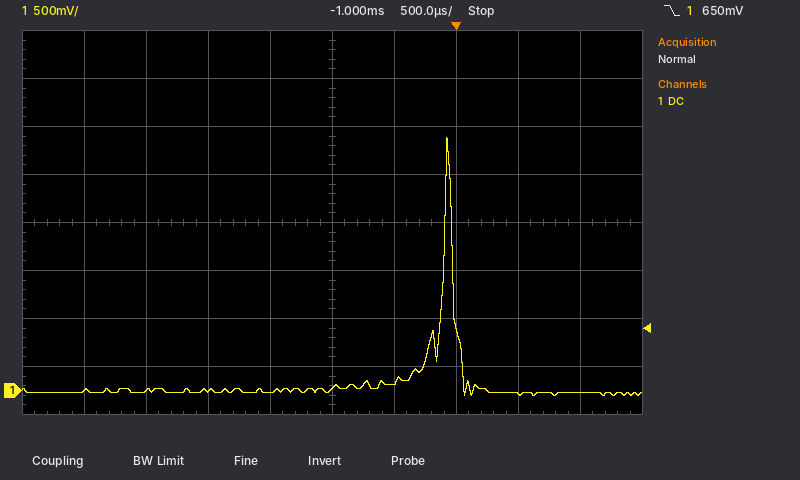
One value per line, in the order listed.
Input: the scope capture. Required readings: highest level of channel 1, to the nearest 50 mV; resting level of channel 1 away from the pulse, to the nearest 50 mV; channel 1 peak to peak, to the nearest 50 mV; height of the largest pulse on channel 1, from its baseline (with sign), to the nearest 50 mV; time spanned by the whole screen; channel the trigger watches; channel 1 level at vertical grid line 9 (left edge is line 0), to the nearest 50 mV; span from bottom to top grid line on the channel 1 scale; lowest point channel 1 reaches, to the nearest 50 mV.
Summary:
2.65 V
0 mV
2.70 V
+2.65 V
5 ms
channel 1
0 mV
4 V
-50 mV
